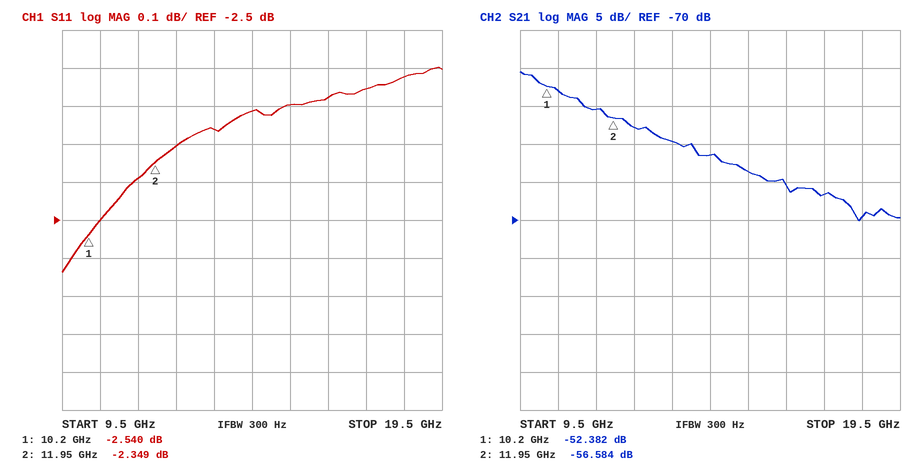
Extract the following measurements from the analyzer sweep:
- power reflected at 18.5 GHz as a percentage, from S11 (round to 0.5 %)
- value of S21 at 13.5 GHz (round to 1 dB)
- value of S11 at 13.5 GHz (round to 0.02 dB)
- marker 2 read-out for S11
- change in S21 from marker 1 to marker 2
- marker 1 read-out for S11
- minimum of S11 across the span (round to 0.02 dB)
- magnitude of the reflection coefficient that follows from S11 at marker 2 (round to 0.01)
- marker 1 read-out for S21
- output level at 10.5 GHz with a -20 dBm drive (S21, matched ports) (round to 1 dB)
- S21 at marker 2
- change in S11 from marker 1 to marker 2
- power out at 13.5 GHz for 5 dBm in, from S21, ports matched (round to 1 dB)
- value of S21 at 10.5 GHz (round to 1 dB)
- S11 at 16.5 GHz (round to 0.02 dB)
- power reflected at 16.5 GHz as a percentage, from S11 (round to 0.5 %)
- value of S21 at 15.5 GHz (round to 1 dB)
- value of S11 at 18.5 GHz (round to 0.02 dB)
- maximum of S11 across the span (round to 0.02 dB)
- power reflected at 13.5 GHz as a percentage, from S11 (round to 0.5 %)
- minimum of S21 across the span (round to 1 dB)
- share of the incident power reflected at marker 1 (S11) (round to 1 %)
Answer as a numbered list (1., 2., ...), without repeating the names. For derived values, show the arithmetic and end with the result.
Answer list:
1. 10^(-2.12/10) ≈ 61.4 %, so 61.5 % to the nearest 0.5 %
2. -60 dB
3. -2.26 dB
4. -2.349 dB
5. -56.584 − (-52.382) = -4.202 dB
6. -2.540 dB
7. -2.64 dB
8. 10^(-2.349/20) ≈ 0.76
9. -52.382 dB
10. -20 dBm + (-53 dB) = -73 dBm
11. -56.584 dB
12. -2.349 − (-2.54) = 0.191 dB
13. 5 dBm + (-60 dB) = -55 dBm
14. -53 dB
15. -2.18 dB
16. 10^(-2.18/10) ≈ 60.5 %
17. -64 dB
18. -2.12 dB
19. -2.10 dB
20. 10^(-2.26/10) ≈ 59.4 %, so 59.5 % to the nearest 0.5 %
21. -70 dB
22. 10^(-2.54/10) ≈ 56 %
